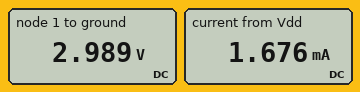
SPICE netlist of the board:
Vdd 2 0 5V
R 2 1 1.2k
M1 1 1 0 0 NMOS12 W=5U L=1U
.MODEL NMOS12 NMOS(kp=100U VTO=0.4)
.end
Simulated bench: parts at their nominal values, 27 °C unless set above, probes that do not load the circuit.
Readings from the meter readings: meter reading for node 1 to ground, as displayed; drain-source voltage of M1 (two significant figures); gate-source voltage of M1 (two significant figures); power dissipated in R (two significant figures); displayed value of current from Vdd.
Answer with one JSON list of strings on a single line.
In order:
["2.989 V", "3.0 V", "3.0 V", "3.4 mW", "1.676 mA"]
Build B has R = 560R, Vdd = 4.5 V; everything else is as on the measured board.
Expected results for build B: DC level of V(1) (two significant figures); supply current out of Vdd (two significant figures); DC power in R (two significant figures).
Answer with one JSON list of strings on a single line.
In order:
["3.3 V", "2.1 mA", "2.5 mW"]
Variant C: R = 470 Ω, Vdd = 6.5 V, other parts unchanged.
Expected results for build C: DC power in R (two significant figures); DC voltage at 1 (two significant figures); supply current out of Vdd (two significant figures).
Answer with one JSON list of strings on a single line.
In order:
["8.4 mW", "4.5 V", "4.2 mA"]
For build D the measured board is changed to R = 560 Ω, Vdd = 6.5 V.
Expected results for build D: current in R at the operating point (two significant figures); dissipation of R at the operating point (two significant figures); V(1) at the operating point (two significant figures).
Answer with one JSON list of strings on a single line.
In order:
["3.9 mA", "8.4 mW", "4.3 V"]
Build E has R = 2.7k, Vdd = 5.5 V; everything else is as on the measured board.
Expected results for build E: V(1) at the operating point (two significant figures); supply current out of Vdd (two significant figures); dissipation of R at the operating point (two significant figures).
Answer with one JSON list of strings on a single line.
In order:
["2.5 V", "1.1 mA", "3.3 mW"]
